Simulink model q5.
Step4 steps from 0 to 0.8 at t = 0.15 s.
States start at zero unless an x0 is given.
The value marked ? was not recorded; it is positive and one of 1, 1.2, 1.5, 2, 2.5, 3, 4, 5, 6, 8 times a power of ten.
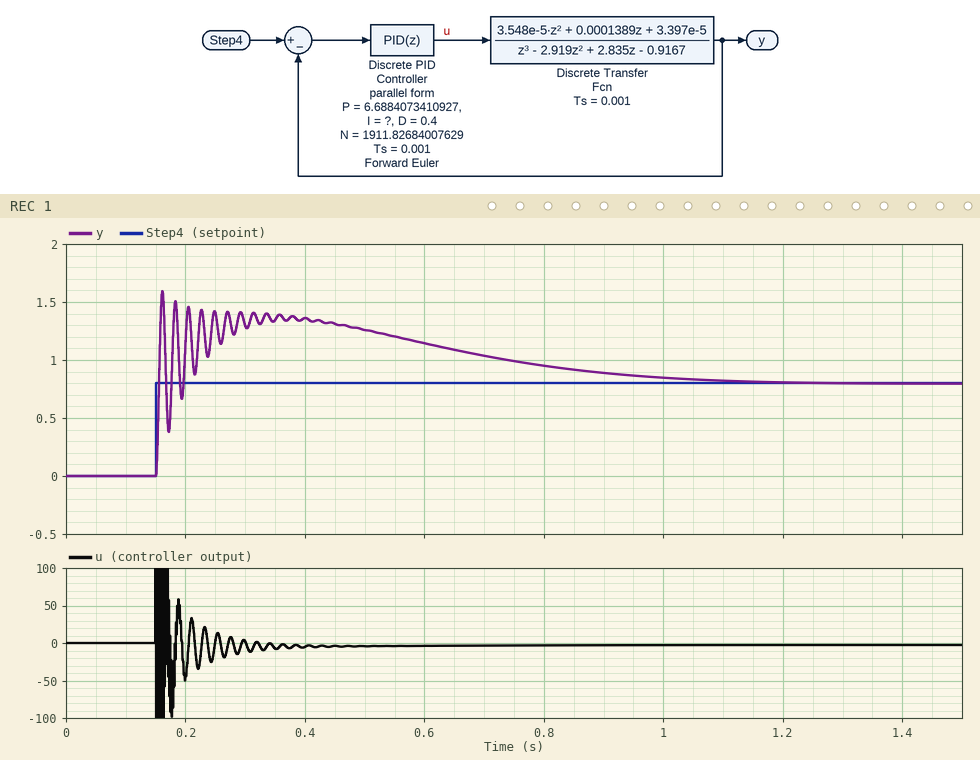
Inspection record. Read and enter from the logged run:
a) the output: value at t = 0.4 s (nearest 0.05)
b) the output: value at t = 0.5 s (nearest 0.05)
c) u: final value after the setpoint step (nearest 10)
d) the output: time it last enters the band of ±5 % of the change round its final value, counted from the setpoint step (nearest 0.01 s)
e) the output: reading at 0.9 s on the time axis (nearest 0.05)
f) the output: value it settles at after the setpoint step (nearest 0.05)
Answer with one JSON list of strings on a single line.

["1.35", "1.25", "0", "0.87 s", "0.90", "0.80"]
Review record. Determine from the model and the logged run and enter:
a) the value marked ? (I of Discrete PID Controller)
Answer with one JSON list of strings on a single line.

["10"]
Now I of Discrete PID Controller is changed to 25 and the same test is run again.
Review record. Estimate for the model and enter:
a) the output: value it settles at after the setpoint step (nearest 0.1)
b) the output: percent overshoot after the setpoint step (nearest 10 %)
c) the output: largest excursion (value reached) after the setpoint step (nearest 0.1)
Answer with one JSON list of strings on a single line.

["0.8", "100 %", "1.6"]
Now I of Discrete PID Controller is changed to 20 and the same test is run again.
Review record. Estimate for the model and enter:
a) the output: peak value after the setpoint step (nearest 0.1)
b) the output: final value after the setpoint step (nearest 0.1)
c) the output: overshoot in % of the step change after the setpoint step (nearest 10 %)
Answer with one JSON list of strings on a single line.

["1.6", "0.8", "100 %"]
